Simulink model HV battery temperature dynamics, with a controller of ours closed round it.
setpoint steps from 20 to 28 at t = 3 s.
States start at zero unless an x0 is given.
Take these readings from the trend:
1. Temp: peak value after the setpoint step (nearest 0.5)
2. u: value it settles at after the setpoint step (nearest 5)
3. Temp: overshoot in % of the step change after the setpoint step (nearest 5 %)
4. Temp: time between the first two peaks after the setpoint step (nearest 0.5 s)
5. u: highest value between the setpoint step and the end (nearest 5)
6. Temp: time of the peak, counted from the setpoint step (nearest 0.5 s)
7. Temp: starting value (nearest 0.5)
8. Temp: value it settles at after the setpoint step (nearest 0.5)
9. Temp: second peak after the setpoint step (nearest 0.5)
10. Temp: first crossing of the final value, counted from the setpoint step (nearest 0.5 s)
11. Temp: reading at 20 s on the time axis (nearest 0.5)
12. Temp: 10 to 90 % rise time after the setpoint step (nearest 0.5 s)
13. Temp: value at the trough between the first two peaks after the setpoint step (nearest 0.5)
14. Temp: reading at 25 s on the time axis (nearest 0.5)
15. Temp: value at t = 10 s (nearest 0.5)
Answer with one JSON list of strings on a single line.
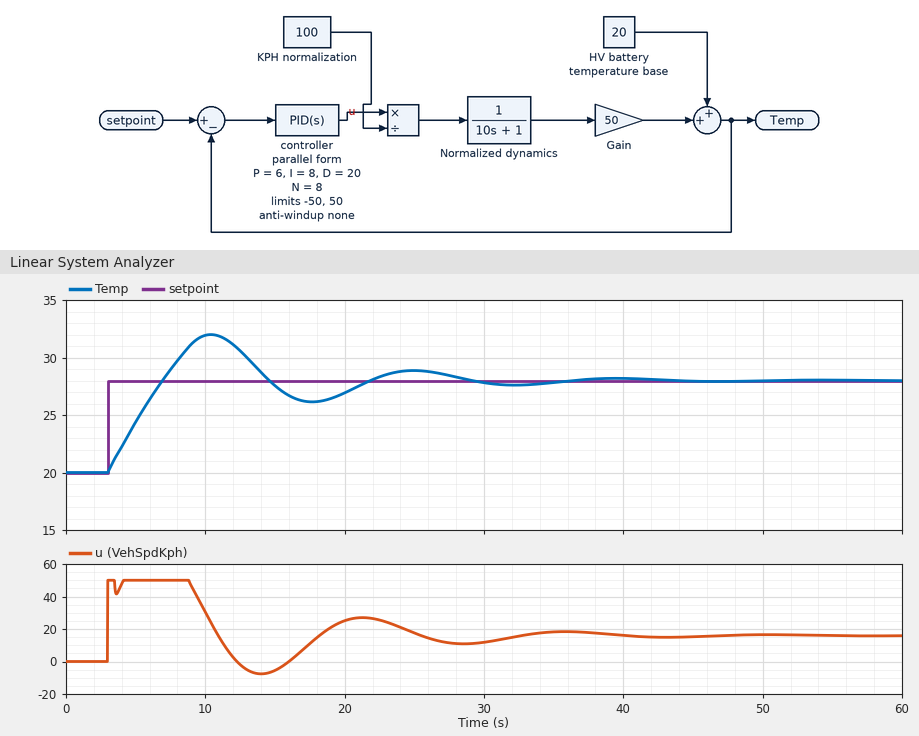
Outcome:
["32.0", "15", "50 %", "14.5 s", "50", "7.5 s", "20.0", "28.0", "29.0", "4.0 s", "27.0", "3.0 s", "26.0", "29.0", "32.0"]
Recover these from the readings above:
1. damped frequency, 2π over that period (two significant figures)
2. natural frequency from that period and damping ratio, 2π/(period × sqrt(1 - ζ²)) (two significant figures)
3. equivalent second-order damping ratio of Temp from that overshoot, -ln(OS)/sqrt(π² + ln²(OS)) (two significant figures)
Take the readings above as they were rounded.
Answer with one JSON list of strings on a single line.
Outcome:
["0.43 rad/s", "0.44 rad/s", "0.22"]
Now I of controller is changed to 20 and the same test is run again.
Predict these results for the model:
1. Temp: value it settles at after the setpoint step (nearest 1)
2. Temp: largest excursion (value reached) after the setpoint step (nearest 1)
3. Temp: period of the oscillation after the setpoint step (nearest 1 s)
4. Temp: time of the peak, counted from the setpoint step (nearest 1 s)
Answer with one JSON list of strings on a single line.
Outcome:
["28", "33", "9 s", "8 s"]
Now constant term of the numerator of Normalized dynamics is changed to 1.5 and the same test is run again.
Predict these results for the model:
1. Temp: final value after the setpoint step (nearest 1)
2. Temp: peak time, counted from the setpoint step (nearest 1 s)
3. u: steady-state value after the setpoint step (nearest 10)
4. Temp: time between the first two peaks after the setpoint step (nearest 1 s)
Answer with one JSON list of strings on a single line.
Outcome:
["28", "6 s", "10", "13 s"]
